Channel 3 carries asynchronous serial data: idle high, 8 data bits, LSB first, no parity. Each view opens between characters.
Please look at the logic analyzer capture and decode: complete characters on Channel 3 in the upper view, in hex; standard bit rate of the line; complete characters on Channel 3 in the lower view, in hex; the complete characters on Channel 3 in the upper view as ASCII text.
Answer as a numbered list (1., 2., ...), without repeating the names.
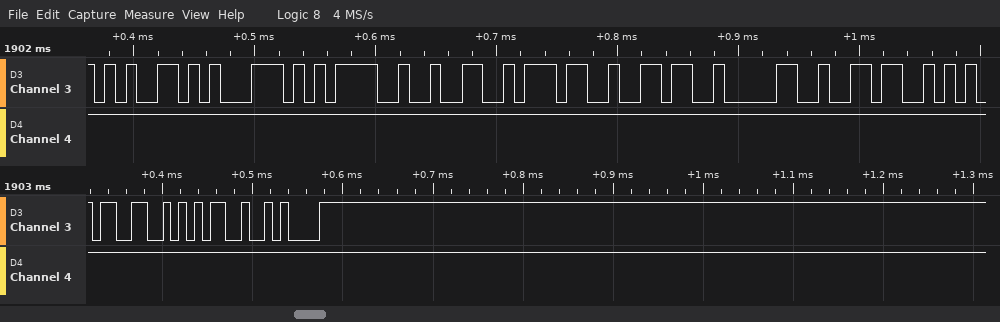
1. 65, 71, 3D, 32, 37, 36, 30, 36
2. 115200 baud
3. 33, 35, 0A
4. "eq=27606"
